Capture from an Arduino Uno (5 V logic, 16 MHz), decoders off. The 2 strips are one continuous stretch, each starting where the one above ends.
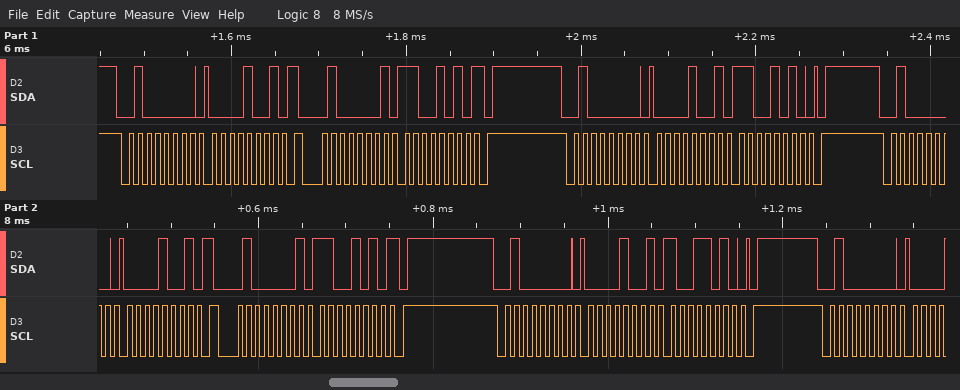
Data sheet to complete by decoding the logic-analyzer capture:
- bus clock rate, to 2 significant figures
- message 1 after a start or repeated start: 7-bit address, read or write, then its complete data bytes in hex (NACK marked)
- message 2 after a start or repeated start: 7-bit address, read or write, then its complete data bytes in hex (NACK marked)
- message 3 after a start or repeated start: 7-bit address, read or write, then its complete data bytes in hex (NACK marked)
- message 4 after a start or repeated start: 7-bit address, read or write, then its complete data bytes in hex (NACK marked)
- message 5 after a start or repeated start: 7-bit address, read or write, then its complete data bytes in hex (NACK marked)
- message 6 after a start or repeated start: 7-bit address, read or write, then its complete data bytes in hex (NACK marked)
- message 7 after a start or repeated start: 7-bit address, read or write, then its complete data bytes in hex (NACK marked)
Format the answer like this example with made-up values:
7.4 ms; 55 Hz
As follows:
100 kHz; 0x20 write: 09; 0x20 read: CA NACK; 0x20 write: 09 CA; 0x20 write: 09; 0x20 read: CA NACK; 0x20 write: 09 9A; 0x20 write
